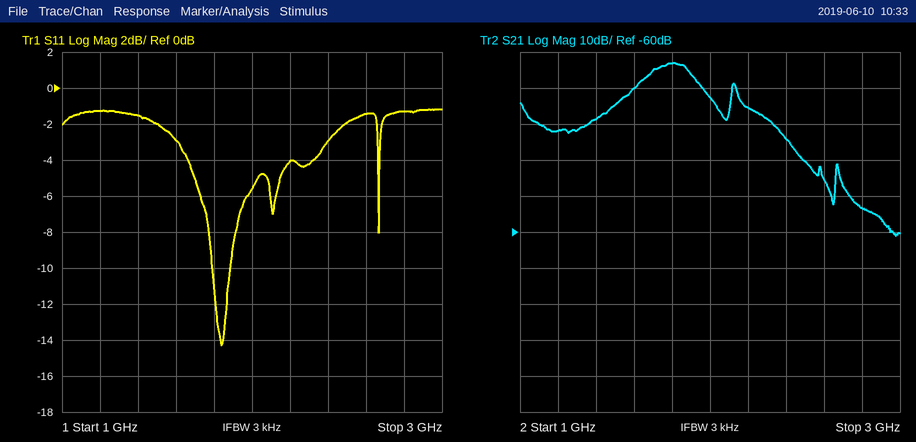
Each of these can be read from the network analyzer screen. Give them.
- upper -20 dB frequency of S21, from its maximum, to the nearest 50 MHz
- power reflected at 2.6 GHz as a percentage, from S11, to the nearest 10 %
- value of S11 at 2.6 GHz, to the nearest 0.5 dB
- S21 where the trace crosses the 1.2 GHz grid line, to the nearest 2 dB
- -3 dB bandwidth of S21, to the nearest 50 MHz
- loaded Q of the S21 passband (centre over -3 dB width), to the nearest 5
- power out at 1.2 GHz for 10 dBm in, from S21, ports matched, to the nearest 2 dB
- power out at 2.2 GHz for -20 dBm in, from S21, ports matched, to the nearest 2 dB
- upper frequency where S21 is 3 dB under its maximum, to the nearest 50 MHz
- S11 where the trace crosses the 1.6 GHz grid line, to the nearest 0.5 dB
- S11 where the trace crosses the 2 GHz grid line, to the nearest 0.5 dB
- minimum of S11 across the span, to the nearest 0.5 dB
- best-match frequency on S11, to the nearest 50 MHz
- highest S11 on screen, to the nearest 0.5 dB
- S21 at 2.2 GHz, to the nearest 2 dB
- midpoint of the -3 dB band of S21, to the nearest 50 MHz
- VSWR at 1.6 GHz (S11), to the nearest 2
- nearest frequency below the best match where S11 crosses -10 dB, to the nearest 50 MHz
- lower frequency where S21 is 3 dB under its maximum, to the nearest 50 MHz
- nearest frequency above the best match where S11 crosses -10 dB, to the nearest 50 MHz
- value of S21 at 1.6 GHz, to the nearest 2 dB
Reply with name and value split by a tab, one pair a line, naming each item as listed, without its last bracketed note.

upper -20 dB frequency of S21, from its maximum, to the nearest 50 MHz	2.40 GHz
power reflected at 2.6 GHz as a percentage, from S11, to the nearest 10 %	70 %
value of S11 at 2.6 GHz, to the nearest 0.5 dB	-1.5 dB
S21 where the trace crosses the 1.2 GHz grid line, to the nearest 2 dB	-32 dB
-3 dB bandwidth of S21, to the nearest 50 MHz	200 MHz
loaded Q of the S21 passband (centre over -3 dB width), to the nearest 5	10
power out at 1.2 GHz for 10 dBm in, from S21, ports matched, to the nearest 2 dB	-22 dBm
power out at 2.2 GHz for -20 dBm in, from S21, ports matched, to the nearest 2 dB	-46 dBm
upper frequency where S21 is 3 dB under its maximum, to the nearest 50 MHz	1.90 GHz
S11 where the trace crosses the 1.6 GHz grid line, to the nearest 0.5 dB	-3.0 dB
S11 where the trace crosses the 2 GHz grid line, to the nearest 0.5 dB	-5.5 dB
minimum of S11 across the span, to the nearest 0.5 dB	-14.5 dB
best-match frequency on S11, to the nearest 50 MHz	1.85 GHz
highest S11 on screen, to the nearest 0.5 dB	-1.0 dB
S21 at 2.2 GHz, to the nearest 2 dB	-26 dB
midpoint of the -3 dB band of S21, to the nearest 50 MHz	1.80 GHz
VSWR at 1.6 GHz (S11), to the nearest 2	6
nearest frequency below the best match where S11 crosses -10 dB, to the nearest 50 MHz	1.80 GHz
lower frequency where S21 is 3 dB under its maximum, to the nearest 50 MHz	1.70 GHz
nearest frequency above the best match where S11 crosses -10 dB, to the nearest 50 MHz	1.90 GHz
value of S21 at 1.6 GHz, to the nearest 2 dB	-20 dB
